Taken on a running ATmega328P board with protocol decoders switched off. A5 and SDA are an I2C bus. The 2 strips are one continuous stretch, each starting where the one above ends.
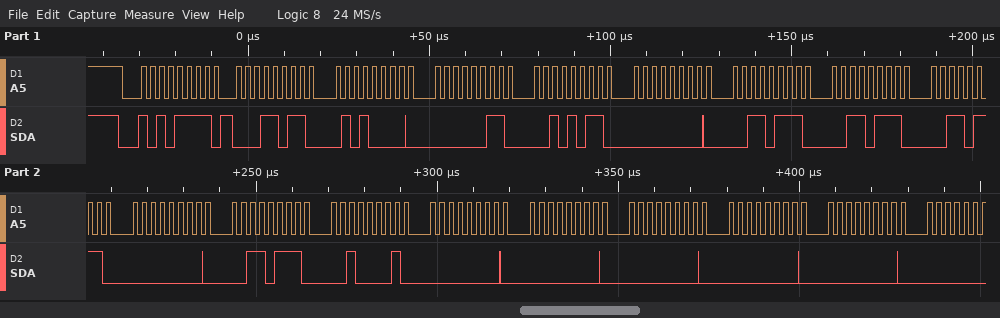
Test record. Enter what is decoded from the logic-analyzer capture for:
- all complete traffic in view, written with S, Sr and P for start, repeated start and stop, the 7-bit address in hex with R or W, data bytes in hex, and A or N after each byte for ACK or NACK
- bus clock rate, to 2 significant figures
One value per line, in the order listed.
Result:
S 57R A 1B A 50 A 03 A 2B A 00 A 37 A 37 A 37 A 00 A 37 A 21 A 00 A 00 A 00 A 00 A 00 A
400 kHz
